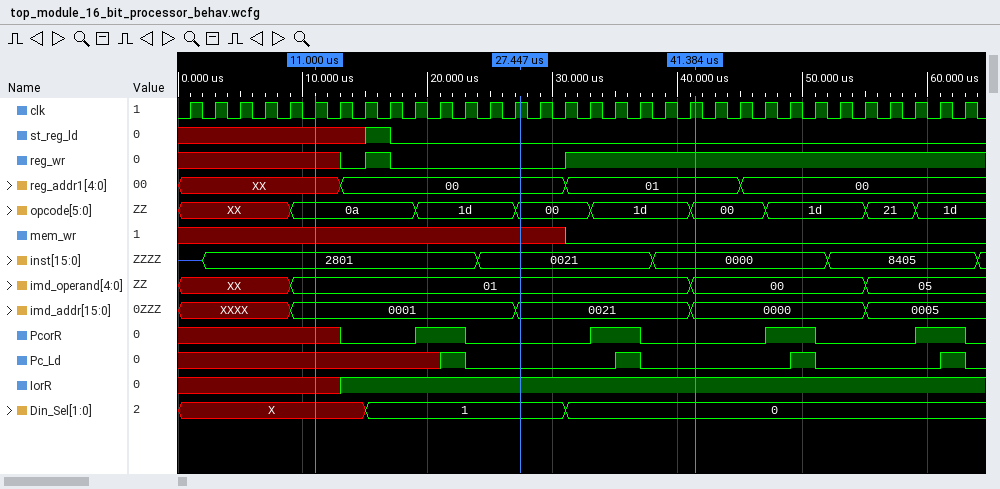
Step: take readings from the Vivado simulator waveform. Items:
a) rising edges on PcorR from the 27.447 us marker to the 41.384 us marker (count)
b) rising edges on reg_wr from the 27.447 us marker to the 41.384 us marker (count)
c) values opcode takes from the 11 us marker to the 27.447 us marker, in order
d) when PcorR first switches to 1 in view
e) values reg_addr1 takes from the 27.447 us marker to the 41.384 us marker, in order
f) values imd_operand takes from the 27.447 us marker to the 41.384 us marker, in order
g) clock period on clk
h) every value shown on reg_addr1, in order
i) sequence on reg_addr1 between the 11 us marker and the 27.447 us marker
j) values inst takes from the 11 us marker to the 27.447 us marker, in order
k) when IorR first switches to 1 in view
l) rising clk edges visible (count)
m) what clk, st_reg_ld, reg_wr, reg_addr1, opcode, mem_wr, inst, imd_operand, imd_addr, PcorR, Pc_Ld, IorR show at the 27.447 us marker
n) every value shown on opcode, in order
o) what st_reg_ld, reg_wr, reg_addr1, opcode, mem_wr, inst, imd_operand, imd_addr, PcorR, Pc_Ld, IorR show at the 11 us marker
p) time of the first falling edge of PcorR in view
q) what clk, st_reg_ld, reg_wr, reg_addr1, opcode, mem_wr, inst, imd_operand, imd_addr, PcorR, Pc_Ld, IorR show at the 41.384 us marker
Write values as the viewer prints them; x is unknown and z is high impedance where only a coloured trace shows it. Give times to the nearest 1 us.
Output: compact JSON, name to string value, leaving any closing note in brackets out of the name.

{"rising edges on PcorR from the 27.447 us marker to the 41.384 us marker": "1", "rising edges on reg_wr from the 27.447 us marker to the 41.384 us marker": "1", "values opcode takes from the 11 us marker to the 27.447 us marker, in order": "0a, 1d, 00", "when PcorR first switches to 1 in view": "19 us", "values reg_addr1 takes from the 27.447 us marker to the 41.384 us marker, in order": "00, 01", "values imd_operand takes from the 27.447 us marker to the 41.384 us marker, in order": "01, 00", "clock period on clk": "2 us", "every value shown on reg_addr1, in order": "XX, 00, 01, 00", "sequence on reg_addr1 between the 11 us marker and the 27.447 us marker": "XX, 00", "values inst takes from the 11 us marker to the 27.447 us marker, in order": "2801, 0021", "when IorR first switches to 1 in view": "13 us", "rising clk edges visible": "32", "what clk, st_reg_ld, reg_wr, reg_addr1, opcode, mem_wr, inst, imd_operand, imd_addr, PcorR, Pc_Ld, IorR show at the 27.447 us marker": "clk=1, st_reg_ld=0, reg_wr=0, reg_addr1=00, opcode=00, mem_wr=x, inst=0021, imd_operand=01, imd_addr=0021, PcorR=0, Pc_Ld=0, IorR=1", "every value shown on opcode, in order": "XX, 0a, 1d, 00, 1d, 00, 1d, 21, 1d", "what st_reg_ld, reg_wr, reg_addr1, opcode, mem_wr, inst, imd_operand, imd_addr, PcorR, Pc_Ld, IorR show at the 11 us marker": "st_reg_ld=x, reg_wr=x, reg_addr1=XX, opcode=0a, mem_wr=x, inst=2801, imd_operand=01, imd_addr=0001, PcorR=x, Pc_Ld=x, IorR=x", "time of the first falling edge of PcorR in view": "23 us", "what clk, st_reg_ld, reg_wr, reg_addr1, opcode, mem_wr, inst, imd_operand, imd_addr, PcorR, Pc_Ld, IorR show at the 41.384 us marker": "clk=1, st_reg_ld=0, reg_wr=1, reg_addr1=01, opcode=00, mem_wr=0, inst=0000, imd_operand=00, imd_addr=0000, PcorR=0, Pc_Ld=0, IorR=1"}
